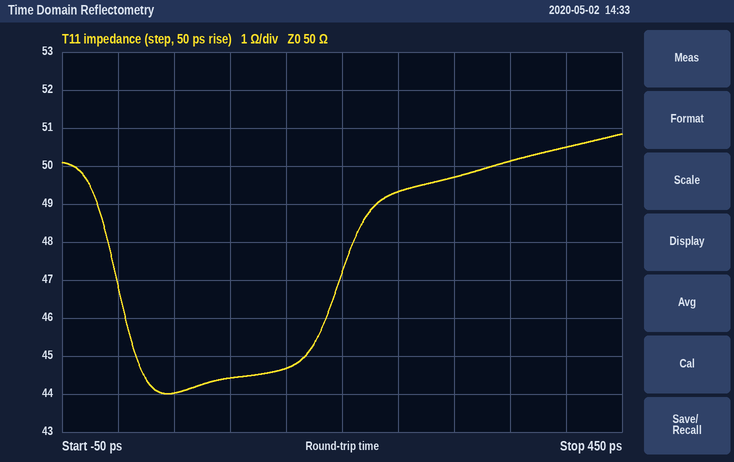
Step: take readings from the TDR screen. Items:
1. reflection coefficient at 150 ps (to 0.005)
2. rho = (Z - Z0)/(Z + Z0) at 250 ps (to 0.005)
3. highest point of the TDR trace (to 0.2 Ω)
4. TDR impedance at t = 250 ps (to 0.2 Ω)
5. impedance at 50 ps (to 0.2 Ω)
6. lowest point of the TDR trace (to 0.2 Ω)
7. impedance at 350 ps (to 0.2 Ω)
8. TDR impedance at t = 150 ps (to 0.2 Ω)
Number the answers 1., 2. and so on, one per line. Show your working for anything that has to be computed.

1. (44.6 − 50)/(44.6 + 50) ≈ -0.0571, so -0.055 to the nearest 0.005
2. (49.4 − 50)/(49.4 + 50) ≈ -0.00604, so -0.005 to the nearest 0.005
3. 50.8 Ω
4. 49.4 Ω
5. 44.0 Ω
6. 44.0 Ω
7. 50.2 Ω
8. 44.6 Ω
